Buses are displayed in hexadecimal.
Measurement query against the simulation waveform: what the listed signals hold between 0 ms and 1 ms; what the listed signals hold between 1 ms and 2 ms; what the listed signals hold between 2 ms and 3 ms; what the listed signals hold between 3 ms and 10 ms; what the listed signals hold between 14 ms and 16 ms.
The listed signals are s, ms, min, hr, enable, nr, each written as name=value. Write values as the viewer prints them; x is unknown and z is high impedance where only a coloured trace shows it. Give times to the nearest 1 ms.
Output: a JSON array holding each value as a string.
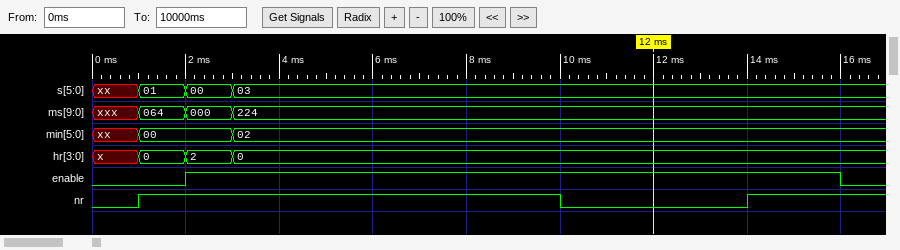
["s=xx, ms=xxx, min=xx, hr=x, enable=0, nr=0", "s=01, ms=064, min=00, hr=0, enable=0, nr=1", "s=00, ms=000, min=00, hr=2, enable=1, nr=1", "s=03, ms=224, min=02, hr=0, enable=1, nr=1", "s=03, ms=224, min=02, hr=0, enable=1, nr=1"]
